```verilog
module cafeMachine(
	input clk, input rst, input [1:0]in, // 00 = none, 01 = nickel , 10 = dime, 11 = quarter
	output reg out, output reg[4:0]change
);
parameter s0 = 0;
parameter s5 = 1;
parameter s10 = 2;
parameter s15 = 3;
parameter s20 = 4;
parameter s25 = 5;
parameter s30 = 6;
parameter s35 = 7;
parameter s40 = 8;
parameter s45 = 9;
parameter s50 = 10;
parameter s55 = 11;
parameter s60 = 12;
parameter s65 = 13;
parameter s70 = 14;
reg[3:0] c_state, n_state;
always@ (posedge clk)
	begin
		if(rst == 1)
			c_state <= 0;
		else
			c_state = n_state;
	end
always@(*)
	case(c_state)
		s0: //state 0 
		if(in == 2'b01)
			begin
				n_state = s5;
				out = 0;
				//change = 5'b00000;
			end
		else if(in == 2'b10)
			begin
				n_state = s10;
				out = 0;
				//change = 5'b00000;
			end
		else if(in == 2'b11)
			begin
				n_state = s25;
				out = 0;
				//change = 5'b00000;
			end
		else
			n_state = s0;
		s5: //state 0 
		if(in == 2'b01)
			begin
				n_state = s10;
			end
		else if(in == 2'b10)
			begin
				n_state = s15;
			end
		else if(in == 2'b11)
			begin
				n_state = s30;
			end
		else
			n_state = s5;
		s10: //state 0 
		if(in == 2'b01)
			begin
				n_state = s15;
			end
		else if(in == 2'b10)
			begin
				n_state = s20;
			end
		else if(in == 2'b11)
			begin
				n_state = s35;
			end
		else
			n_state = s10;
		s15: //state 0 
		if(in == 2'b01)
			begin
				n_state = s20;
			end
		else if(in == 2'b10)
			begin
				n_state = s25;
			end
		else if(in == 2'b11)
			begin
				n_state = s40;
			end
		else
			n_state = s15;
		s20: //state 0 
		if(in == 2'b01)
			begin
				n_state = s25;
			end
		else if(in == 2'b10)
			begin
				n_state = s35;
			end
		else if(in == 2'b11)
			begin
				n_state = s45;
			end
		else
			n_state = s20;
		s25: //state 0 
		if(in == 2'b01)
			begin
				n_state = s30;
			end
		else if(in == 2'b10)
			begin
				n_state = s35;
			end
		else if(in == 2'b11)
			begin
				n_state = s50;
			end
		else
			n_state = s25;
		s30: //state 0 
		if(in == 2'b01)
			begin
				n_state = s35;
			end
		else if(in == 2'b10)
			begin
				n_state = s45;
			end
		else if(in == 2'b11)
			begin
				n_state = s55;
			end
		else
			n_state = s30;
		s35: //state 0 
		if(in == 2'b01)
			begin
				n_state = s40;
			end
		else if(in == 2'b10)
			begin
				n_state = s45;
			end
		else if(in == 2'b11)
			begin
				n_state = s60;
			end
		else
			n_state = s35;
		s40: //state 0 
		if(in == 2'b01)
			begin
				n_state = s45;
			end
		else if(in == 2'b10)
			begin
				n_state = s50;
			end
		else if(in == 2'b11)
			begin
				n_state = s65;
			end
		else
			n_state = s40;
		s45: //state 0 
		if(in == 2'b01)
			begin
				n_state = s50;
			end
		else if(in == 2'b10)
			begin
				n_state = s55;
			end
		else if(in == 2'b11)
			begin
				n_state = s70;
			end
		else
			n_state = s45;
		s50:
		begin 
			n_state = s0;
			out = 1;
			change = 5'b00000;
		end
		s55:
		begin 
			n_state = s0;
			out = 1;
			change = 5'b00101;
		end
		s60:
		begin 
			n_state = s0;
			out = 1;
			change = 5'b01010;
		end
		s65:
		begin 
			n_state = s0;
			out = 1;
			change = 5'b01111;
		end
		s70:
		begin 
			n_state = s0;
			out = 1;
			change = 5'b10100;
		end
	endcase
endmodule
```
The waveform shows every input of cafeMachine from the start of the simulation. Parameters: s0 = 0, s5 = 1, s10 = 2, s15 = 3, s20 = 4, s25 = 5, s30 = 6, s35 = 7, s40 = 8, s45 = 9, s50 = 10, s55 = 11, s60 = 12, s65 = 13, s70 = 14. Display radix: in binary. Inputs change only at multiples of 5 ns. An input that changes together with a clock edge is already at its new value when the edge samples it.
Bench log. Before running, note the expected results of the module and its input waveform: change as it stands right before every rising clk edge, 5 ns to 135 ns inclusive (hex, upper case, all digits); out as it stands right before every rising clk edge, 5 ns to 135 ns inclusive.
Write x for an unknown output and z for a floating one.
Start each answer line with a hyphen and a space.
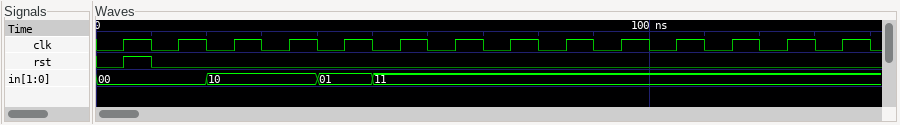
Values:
- x, x, x, x, x, x, 00, 00, 00, 00, 00, 00, 00, 00
- x x 0 0 0 0 1 0 0 1 0 0 1 0
